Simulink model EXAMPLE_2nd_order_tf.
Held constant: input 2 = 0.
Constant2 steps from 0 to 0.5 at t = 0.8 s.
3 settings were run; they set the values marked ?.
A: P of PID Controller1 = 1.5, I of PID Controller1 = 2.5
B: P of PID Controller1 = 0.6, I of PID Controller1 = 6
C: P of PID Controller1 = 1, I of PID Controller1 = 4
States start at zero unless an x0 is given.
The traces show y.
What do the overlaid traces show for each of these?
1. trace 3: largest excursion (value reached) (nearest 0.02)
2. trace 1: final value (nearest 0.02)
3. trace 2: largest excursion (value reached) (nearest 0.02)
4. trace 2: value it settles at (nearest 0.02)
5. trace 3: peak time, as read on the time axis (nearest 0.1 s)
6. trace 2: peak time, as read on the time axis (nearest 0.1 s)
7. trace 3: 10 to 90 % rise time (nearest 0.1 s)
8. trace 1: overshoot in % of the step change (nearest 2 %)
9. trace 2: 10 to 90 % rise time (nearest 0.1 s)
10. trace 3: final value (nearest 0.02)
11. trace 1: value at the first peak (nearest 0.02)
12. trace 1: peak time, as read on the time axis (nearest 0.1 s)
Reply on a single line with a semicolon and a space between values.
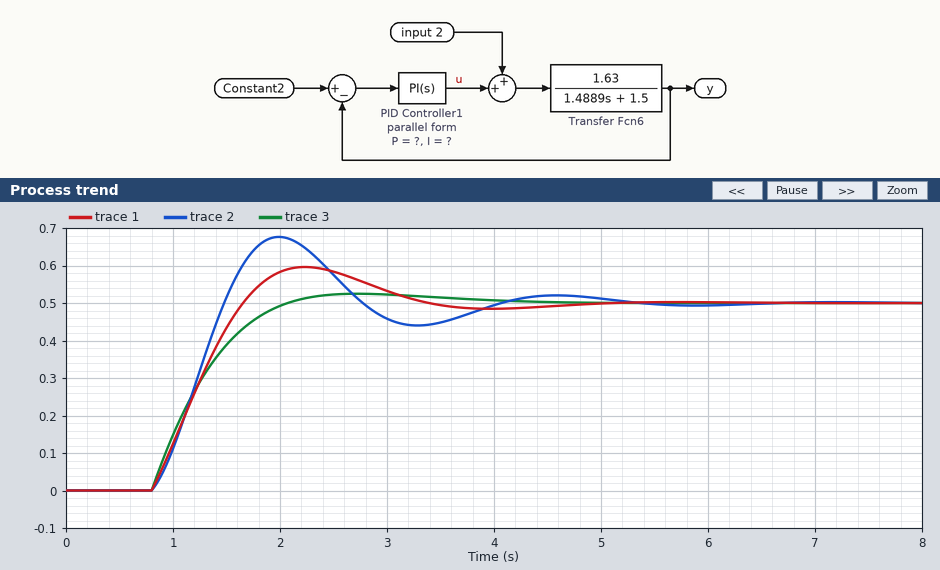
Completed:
0.52; 0.50; 0.68; 0.50; 2.7 s; 2.0 s; 0.9 s; 20 %; 0.5 s; 0.50; 0.60; 2.2 s
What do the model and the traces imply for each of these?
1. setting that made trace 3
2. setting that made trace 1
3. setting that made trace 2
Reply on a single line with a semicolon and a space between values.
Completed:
A; C; B
